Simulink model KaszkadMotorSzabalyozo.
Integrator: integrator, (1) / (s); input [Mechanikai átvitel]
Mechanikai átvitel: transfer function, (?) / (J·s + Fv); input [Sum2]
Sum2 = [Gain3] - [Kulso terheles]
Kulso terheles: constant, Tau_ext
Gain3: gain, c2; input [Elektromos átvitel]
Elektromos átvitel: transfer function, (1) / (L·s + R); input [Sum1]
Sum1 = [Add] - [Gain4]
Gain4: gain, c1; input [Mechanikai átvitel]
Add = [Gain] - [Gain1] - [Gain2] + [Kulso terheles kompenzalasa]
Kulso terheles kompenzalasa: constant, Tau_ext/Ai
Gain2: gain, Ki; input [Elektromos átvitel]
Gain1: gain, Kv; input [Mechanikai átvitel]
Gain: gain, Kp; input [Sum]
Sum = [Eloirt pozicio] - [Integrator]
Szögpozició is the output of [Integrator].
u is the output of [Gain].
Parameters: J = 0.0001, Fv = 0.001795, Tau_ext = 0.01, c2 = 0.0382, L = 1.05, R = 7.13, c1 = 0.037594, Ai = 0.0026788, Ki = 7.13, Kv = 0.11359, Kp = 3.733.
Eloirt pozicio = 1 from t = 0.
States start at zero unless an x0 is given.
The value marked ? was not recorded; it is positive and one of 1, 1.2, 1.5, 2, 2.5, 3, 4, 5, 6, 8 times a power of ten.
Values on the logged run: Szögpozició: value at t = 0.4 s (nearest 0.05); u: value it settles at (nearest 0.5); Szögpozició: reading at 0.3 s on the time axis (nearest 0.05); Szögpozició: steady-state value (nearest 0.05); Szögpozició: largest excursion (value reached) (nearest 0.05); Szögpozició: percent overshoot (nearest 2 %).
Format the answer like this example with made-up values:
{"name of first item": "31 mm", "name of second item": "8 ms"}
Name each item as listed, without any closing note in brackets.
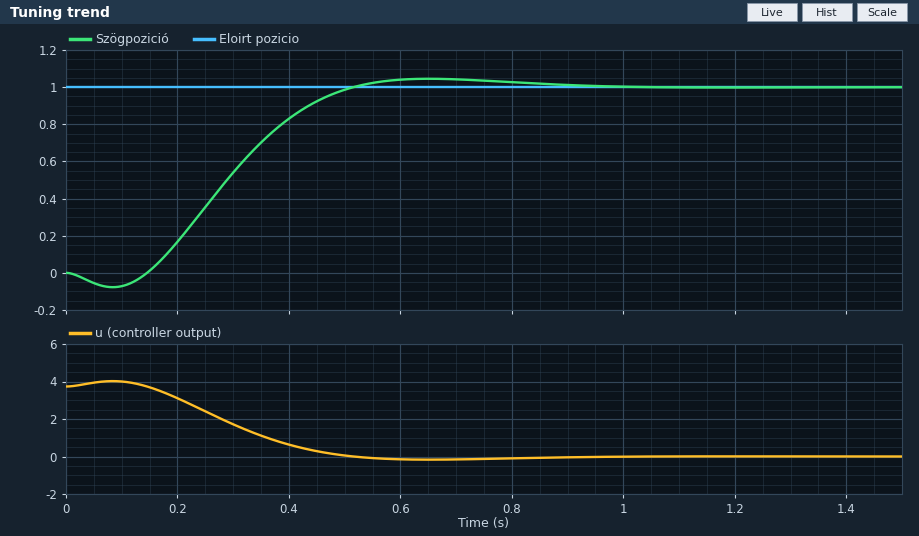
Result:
{"Szögpozició: value at t = 0.4 s": "0.85", "u: value it settles at": "0.0", "Szögpozició: reading at 0.3 s on the time axis": "0.55", "Szögpozició: steady-state value": "1.00", "Szögpozició: largest excursion (value reached)": "1.05", "Szögpozició: percent overshoot": "4 %"}
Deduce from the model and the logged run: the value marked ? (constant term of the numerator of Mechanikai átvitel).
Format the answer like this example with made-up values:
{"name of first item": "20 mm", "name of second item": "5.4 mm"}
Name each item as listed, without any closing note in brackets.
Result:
{"the value marked ?": "1"}
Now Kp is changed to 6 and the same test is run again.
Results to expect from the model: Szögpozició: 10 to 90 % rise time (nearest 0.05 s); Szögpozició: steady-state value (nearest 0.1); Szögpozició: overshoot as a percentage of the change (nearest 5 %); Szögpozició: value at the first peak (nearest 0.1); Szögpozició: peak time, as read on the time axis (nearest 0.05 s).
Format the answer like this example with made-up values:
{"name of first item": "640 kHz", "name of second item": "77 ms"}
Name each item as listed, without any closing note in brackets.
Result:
{"Szögpozició: 10 to 90 % rise time": "0.15 s", "Szögpozició: steady-state value": "1.0", "Szögpozició: overshoot as a percentage of the change": "20 %", "Szögpozició: value at the first peak": "1.2", "Szögpozició: peak time, as read on the time axis": "0.45 s"}
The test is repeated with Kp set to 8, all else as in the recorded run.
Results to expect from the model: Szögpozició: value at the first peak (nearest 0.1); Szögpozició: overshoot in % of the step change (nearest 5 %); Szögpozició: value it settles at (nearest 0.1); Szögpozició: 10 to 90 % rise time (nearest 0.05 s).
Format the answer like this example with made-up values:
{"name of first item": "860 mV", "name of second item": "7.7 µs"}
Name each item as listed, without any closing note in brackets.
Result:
{"Szögpozició: value at the first peak": "1.3", "Szögpozició: overshoot in % of the step change": "30 %", "Szögpozició: value it settles at": "1.0", "Szögpozició: 10 to 90 % rise time": "0.15 s"}
